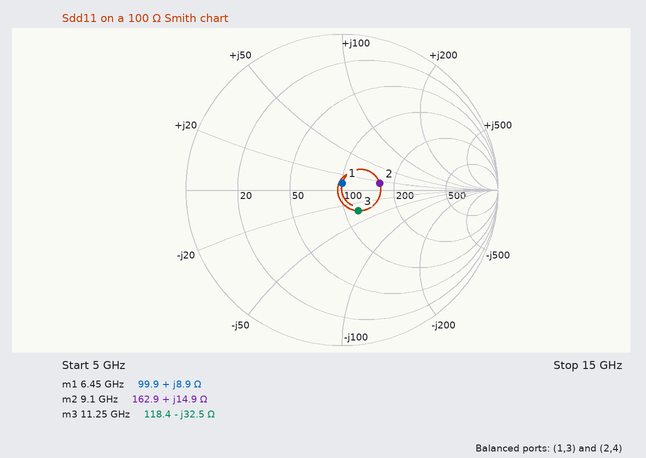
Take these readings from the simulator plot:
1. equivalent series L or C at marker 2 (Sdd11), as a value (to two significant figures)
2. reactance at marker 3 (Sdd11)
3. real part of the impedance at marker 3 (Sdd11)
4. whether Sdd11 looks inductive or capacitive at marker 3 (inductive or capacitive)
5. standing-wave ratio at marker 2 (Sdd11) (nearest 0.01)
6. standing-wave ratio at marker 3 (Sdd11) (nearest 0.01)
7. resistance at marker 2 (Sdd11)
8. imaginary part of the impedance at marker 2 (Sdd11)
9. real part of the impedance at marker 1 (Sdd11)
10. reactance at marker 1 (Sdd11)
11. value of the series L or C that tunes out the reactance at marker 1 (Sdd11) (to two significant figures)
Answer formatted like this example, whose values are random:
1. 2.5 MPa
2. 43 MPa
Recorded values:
1. 260 pH
2. -32.5 Ω
3. 118.4 Ω
4. capacitive
5. 1.65
6. 1.41
7. 162.9 Ω
8. +14.9 Ω
9. 99.9 Ω
10. +8.9 Ω
11. 2.8 pF
